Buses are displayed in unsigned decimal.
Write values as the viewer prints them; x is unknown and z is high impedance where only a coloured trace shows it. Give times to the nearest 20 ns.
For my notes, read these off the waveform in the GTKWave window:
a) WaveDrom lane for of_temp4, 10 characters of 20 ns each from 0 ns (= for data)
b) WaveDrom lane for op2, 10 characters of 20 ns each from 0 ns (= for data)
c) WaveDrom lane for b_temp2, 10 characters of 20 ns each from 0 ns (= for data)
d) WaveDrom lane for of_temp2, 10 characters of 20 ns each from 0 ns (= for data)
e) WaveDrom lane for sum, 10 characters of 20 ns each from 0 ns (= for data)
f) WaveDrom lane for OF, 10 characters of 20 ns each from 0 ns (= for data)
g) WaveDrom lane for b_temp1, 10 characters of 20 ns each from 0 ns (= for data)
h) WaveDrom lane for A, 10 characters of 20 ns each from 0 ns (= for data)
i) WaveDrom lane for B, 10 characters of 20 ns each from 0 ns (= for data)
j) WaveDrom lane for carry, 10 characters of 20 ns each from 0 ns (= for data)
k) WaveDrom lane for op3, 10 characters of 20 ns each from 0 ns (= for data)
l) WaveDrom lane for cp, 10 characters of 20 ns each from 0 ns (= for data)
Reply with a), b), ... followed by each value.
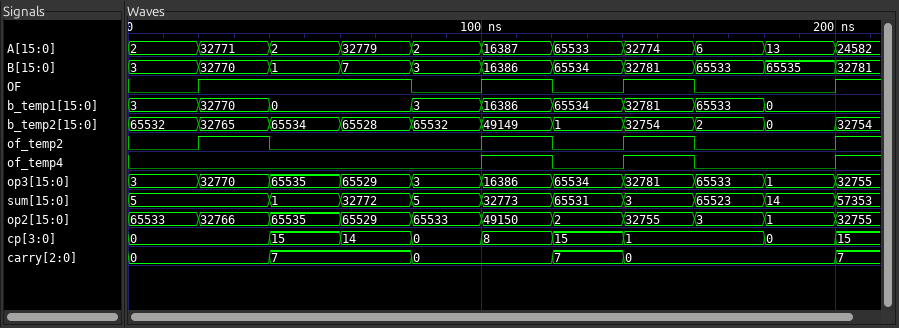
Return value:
a) {name: 'of_temp4', wave: '0....1010.'}
b) {name: 'op2', wave: '==========', data: '65533 32766 65535 65529 65533 49150 2 32755 3 1'}
c) {name: 'b_temp2', wave: '==========', data: '65532 32765 65534 65528 65532 49149 1 32754 2 0'}
d) {name: 'of_temp2', wave: '010..1010.'}
e) {name: 'sum', wave: '=.========', data: '5 1 32772 5 32773 65531 3 65523 14'}
f) {name: 'OF', wave: '01..01010.'}
g) {name: 'b_temp1', wave: '===.======', data: '3 32770 0 3 16386 65534 32781 65533 0'}
h) {name: 'A', wave: '==========', data: '2 32771 2 32779 2 16387 65533 32774 6 13'}
i) {name: 'B', wave: '==========', data: '3 32770 1 7 3 16386 65534 32781 65533 65535'}
j) {name: 'carry', wave: '=.=.=.==..', data: '0 7 0 7 0'}
k) {name: 'op3', wave: '==========', data: '3 32770 65535 65529 3 16386 65534 32781 65533 1'}
l) {name: 'cp', wave: '=.======.=', data: '0 15 14 0 8 15 1 0'}
